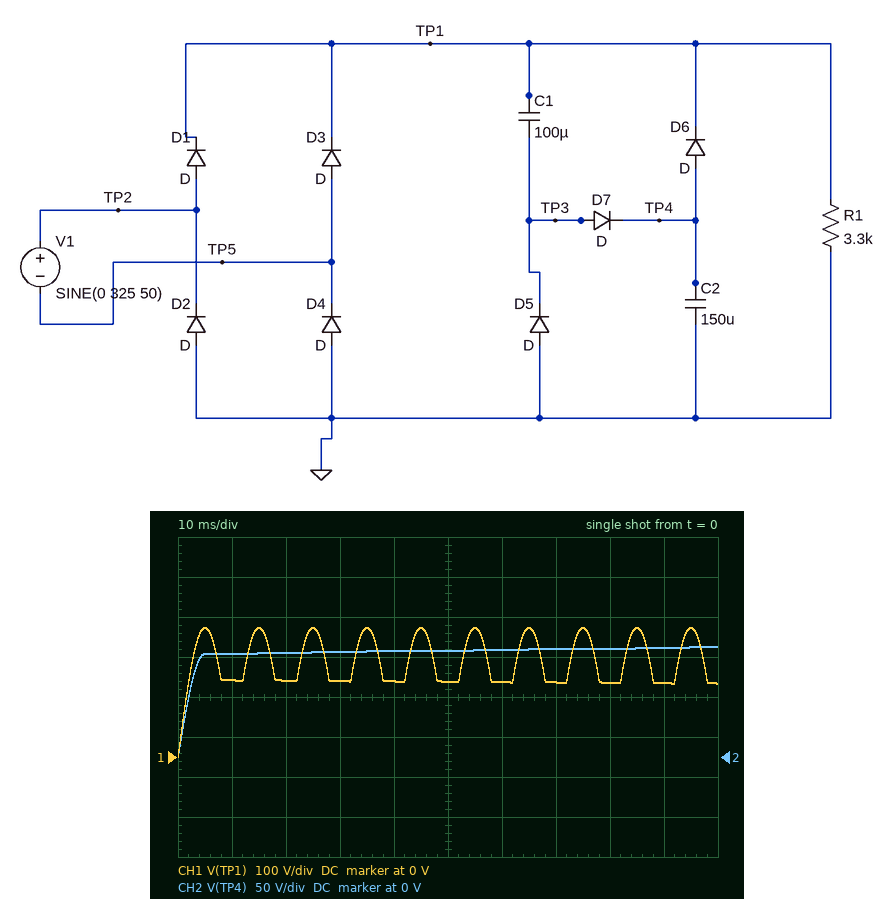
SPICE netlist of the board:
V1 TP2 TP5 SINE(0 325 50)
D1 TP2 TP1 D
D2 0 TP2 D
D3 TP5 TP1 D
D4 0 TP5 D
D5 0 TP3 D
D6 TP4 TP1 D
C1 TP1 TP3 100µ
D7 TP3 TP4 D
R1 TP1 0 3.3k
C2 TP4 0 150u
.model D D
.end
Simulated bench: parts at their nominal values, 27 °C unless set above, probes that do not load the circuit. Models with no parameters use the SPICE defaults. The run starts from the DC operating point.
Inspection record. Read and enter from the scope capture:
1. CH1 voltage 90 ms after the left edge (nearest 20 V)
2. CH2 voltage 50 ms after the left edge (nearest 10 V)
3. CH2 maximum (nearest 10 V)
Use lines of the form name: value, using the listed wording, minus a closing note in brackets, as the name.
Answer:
CH1 voltage 90 ms after the left edge: 180 V
CH2 voltage 50 ms after the left edge: 130 V
CH2 maximum: 140 V
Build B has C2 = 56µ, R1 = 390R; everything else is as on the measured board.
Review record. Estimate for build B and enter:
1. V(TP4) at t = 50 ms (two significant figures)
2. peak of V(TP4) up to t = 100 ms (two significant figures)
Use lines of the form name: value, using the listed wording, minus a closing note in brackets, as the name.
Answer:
V(TP4) at t = 50 ms: 160 V
peak of V(TP4) up to t = 100 ms: 210 V
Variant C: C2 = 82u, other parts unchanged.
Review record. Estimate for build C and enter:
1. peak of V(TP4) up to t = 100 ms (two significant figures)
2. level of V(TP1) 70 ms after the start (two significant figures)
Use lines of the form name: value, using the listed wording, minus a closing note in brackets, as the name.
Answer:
peak of V(TP4) up to t = 100 ms: 180 V
level of V(TP1) 70 ms after the start: 170 V
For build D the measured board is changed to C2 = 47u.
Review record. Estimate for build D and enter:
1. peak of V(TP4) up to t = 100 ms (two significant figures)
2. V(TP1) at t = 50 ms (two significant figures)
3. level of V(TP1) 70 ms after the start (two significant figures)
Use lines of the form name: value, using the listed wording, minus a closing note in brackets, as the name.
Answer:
peak of V(TP4) up to t = 100 ms: 220 V
V(TP1) at t = 50 ms: 210 V
level of V(TP1) 70 ms after the start: 200 V
